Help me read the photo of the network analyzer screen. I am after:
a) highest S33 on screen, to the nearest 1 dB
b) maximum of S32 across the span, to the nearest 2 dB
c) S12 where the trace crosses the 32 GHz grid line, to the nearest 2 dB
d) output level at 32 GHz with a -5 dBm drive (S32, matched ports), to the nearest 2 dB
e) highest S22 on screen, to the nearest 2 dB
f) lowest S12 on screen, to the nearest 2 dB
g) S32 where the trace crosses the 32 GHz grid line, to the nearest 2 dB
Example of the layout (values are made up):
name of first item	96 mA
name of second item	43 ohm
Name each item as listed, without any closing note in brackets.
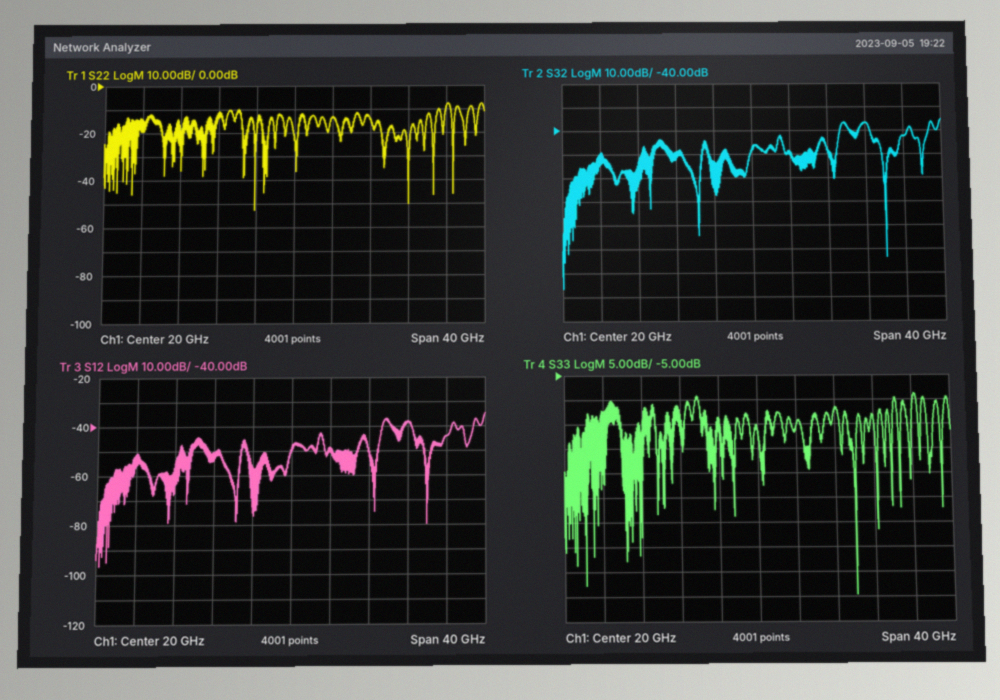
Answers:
highest S33 on screen, to the nearest 1 dB	-9 dB
maximum of S32 across the span, to the nearest 2 dB	-36 dB
S12 where the trace crosses the 32 GHz grid line, to the nearest 2 dB	-38 dB
output level at 32 GHz with a -5 dBm drive (S32, matched ports), to the nearest 2 dB	-42 dBm
highest S22 on screen, to the nearest 2 dB	-8 dB
lowest S12 on screen, to the nearest 2 dB	-96 dB
S32 where the trace crosses the 32 GHz grid line, to the nearest 2 dB	-36 dB
